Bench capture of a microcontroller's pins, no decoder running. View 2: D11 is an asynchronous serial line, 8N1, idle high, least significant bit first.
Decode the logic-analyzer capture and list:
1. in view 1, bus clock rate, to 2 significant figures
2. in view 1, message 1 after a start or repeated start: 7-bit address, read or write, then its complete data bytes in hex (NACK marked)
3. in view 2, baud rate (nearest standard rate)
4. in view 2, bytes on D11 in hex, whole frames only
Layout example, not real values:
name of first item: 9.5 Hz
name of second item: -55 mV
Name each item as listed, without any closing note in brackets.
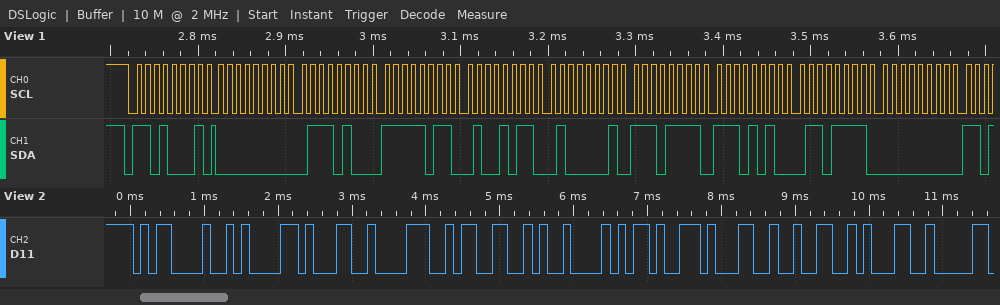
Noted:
in view 1, bus clock rate, to 2 significant figures: 100 kHz
in view 1, message 1 after a start or repeated start: 7-bit address, read or write, then its complete data bytes in hex: 0x68 read: 00 74 FB 4B 41 EF EA 6F 00
in view 2, baud rate: 9600 baud
in view 2, bytes on D11 in hex, whole frames only: 0x0D 0x0A 0x31 0x38 0x33 0x09 0x2D 0x31 0x32 0x31
